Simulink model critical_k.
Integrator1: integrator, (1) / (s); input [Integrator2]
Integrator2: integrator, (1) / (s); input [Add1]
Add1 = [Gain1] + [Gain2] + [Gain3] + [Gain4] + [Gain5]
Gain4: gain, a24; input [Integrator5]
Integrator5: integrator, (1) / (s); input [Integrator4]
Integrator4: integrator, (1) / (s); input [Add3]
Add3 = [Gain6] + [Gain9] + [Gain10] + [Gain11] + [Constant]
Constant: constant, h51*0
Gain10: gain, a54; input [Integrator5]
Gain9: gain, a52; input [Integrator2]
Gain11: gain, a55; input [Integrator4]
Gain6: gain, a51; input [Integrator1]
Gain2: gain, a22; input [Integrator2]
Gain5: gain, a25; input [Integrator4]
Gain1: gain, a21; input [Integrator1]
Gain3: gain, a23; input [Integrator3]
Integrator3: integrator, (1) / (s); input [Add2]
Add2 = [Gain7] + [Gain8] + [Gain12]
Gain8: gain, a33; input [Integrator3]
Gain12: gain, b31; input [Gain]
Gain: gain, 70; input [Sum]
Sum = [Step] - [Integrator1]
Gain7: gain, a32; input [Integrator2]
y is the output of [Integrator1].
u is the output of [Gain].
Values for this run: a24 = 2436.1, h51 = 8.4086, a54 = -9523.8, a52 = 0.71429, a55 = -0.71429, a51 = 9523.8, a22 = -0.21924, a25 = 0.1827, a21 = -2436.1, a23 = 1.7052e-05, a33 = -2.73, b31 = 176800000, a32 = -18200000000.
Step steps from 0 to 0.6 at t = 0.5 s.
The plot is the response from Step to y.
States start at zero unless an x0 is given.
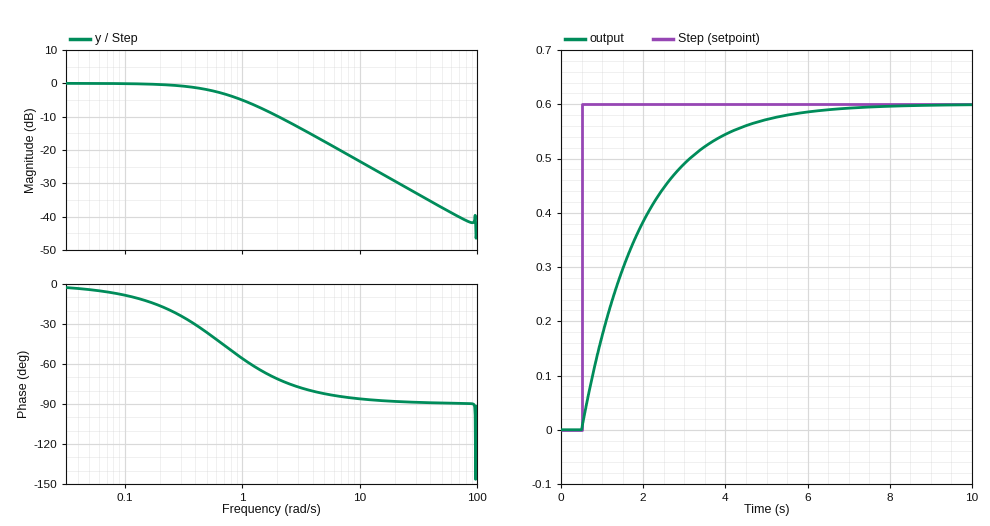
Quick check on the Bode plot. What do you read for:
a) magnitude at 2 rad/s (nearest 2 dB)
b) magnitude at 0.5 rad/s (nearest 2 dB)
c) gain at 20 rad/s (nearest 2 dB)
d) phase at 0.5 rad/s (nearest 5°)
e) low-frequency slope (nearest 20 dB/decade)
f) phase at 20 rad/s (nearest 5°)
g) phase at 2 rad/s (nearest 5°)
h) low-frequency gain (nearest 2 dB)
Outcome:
-10 dB
-2 dB
-30 dB
-35°
0 dB/decade
-90°
-70°
0 dB
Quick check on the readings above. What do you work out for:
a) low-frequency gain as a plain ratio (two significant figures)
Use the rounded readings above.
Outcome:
1.0
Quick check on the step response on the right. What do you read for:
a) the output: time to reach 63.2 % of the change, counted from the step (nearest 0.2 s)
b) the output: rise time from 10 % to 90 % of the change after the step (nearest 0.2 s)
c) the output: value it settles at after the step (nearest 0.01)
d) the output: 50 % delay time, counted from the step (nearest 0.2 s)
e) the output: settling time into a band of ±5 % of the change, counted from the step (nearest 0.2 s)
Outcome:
1.4 s
3.2 s
0.60
1.0 s
4.4 s
